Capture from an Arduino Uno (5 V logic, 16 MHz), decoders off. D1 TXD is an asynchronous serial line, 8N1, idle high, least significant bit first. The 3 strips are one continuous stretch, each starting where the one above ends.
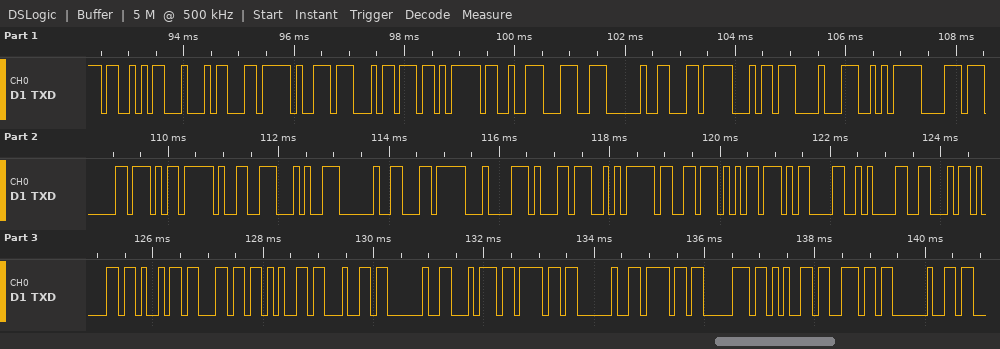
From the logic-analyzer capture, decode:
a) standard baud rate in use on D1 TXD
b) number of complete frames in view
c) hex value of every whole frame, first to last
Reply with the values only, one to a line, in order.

9600 baud
42
53 44 EC B9 B4 EB 93 9C 20 EC B4 88 EA B8 B0 ED 99 94 20 EC 84 B1 EA B3 B5 0D 0A 46 61 69 6C 65 64 20 74 6F 20 6F 70 65 6E 20
